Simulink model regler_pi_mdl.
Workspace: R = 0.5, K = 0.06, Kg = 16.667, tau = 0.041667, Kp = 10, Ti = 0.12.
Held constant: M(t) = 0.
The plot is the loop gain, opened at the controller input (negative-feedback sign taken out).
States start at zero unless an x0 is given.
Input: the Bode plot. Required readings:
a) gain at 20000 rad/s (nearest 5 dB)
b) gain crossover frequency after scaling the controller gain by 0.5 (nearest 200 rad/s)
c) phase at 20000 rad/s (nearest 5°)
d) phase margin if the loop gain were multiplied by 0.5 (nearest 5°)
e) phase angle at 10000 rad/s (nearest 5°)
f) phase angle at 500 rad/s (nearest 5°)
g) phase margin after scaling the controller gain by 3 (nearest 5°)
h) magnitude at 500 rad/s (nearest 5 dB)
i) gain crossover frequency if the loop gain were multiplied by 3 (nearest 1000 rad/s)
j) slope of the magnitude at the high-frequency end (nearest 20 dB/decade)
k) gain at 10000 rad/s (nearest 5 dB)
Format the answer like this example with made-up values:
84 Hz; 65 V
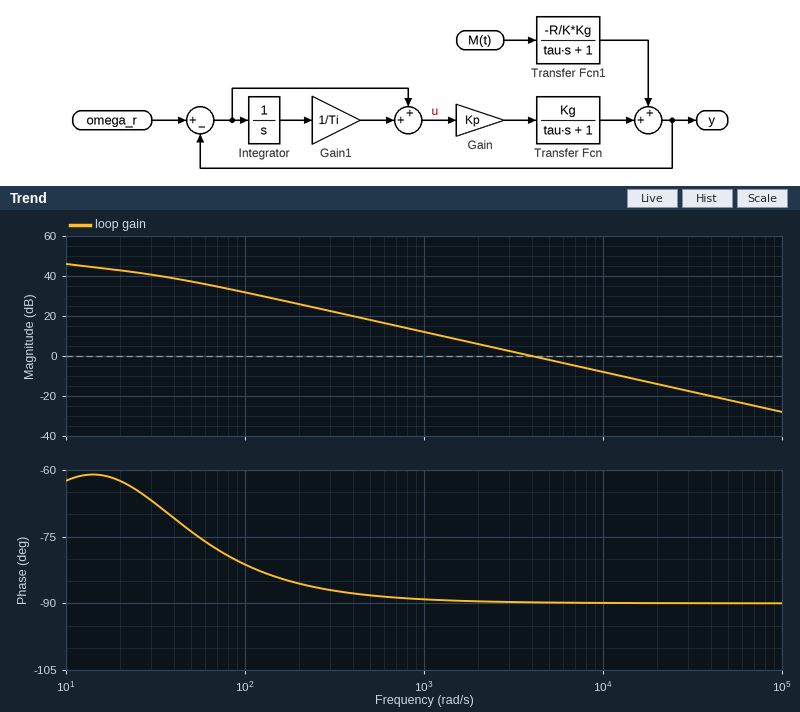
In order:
-15 dB; 2000 rad/s; -90°; 90°; -90°; -90°; 90°; 20 dB; 12000 rad/s; -20 dB/decade; -10 dB
